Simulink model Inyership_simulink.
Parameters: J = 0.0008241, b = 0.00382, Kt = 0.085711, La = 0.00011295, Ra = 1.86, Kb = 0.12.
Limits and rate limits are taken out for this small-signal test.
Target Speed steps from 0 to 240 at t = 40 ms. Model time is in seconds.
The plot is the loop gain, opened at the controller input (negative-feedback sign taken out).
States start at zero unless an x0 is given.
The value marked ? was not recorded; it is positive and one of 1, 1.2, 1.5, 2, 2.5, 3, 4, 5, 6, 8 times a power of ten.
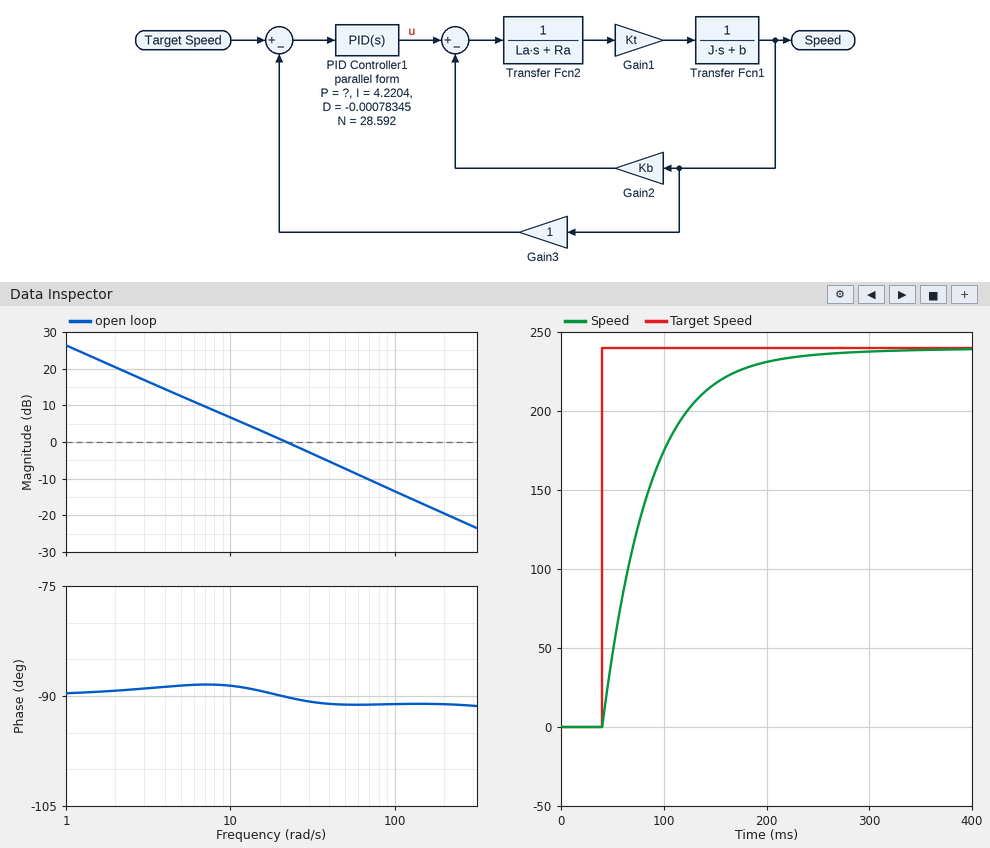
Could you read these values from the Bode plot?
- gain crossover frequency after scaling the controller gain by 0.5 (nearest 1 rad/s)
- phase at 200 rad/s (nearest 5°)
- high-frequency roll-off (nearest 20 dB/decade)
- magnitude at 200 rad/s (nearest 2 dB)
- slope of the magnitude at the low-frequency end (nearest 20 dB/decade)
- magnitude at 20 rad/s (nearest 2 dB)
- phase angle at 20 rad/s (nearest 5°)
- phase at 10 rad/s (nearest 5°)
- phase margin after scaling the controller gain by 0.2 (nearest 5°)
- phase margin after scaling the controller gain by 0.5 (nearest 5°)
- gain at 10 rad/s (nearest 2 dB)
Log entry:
11 rad/s
-90°
-20 dB/decade
-20 dB
-20 dB/decade
0 dB
-90°
-90°
90°
90°
6 dB
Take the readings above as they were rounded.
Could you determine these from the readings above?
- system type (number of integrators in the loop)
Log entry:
1
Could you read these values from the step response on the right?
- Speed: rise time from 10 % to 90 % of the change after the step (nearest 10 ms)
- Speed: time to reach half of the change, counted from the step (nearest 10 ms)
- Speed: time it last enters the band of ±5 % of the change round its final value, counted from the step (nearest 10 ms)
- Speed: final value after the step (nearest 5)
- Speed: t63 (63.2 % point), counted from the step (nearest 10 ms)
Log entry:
100 ms
30 ms
140 ms
240
50 ms
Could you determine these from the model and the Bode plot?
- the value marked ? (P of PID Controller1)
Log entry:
0.4
